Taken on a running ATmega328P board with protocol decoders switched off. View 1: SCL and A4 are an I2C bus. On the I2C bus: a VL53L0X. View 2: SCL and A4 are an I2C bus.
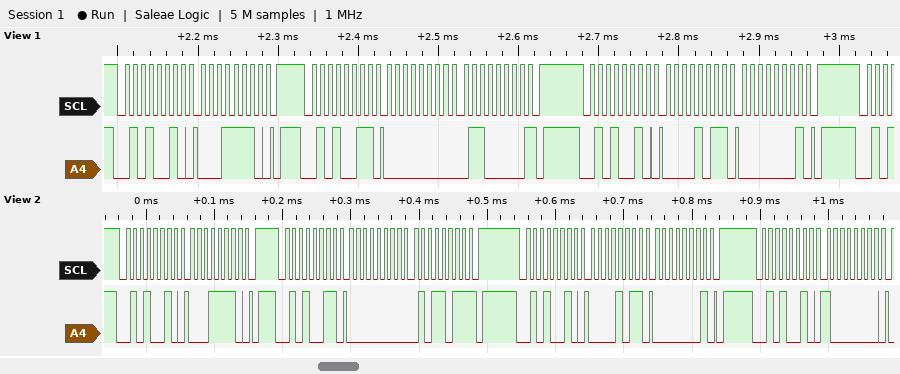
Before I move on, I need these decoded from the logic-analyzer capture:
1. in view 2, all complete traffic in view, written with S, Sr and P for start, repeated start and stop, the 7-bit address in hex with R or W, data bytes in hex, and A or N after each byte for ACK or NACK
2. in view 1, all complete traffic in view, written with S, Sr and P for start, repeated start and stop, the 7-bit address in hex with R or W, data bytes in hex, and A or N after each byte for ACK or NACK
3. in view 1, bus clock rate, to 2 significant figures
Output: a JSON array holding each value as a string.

["S 29W A 1E A P S 29R A 00 A 5B N P S 29W A 0B A 01 A P S 29W A 80 A", "S 29W A 1E A P S 29R A 00 A 60 N P S 29W A 0B A 01 A P", "100 kHz"]
